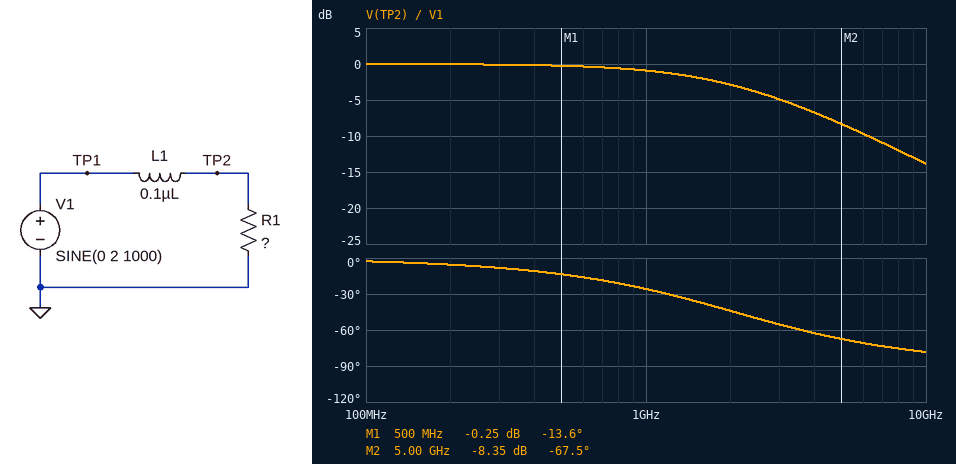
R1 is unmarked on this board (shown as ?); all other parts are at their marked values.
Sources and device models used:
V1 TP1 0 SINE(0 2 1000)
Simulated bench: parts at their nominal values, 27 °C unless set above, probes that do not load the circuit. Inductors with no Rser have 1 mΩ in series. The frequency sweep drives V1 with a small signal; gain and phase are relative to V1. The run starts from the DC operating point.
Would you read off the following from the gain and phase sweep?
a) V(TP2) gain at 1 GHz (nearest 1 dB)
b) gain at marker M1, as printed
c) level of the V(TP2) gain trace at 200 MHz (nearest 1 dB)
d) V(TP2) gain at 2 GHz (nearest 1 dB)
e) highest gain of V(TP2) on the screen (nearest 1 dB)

-1 dB
-0.25 dB
0 dB
-3 dB
0 dB
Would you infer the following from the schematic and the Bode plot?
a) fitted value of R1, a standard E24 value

1.3 kΩ
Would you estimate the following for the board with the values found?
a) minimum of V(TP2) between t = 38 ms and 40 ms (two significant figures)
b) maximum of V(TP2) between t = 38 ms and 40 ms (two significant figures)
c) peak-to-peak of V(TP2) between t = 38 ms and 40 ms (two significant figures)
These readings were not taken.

-2.0 V
2.0 V
4.0 V
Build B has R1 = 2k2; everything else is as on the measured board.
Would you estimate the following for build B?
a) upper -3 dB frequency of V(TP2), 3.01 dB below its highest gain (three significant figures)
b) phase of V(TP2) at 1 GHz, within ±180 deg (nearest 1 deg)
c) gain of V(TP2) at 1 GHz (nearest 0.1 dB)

3.50 GHz
-16 deg
-0.3 dB
